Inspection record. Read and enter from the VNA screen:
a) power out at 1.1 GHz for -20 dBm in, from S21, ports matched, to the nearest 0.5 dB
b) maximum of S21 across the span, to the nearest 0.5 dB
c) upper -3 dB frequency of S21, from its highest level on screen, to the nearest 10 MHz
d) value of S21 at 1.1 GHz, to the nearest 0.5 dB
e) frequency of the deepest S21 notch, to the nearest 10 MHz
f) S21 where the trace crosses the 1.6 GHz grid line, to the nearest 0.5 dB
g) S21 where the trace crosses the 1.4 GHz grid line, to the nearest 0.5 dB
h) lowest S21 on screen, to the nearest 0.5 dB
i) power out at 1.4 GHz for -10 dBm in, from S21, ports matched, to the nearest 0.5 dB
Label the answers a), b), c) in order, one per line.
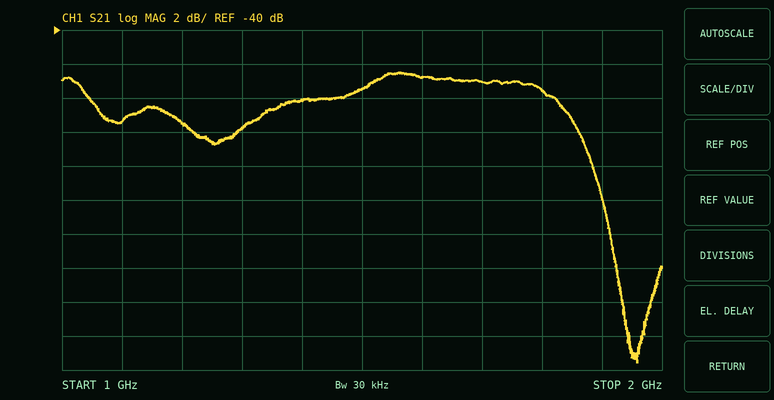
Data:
a) -65.5 dBm
b) -42.5 dB
c) 1.85 GHz
d) -45.5 dB
e) 1.96 GHz
f) -43.0 dB
g) -44.0 dB
h) -59.5 dB
i) -54.0 dBm
